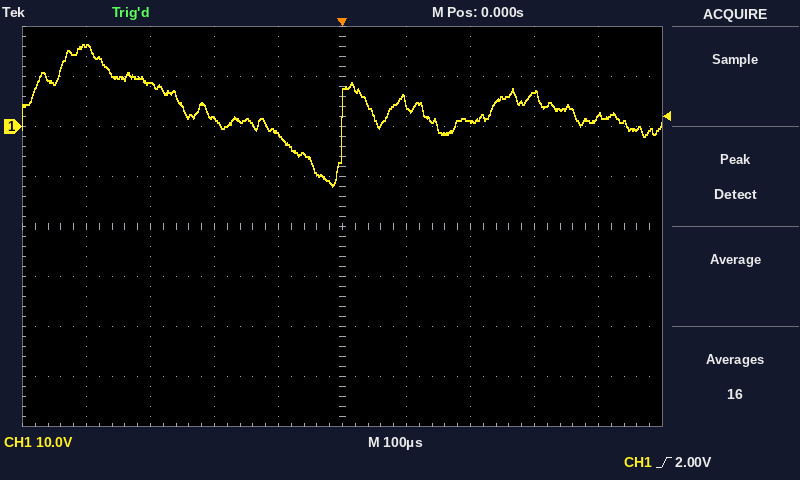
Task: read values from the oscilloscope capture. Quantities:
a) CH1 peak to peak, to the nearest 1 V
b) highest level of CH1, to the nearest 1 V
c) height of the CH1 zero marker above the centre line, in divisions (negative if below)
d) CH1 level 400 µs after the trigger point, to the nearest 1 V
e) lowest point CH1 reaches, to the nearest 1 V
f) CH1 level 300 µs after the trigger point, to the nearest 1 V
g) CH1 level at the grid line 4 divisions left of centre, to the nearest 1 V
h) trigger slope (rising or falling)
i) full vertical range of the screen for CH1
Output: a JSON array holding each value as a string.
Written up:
["28 V", "16 V", "+2.0 div", "2 V", "-12 V", "7 V", "16 V", "rising", "80 V"]
